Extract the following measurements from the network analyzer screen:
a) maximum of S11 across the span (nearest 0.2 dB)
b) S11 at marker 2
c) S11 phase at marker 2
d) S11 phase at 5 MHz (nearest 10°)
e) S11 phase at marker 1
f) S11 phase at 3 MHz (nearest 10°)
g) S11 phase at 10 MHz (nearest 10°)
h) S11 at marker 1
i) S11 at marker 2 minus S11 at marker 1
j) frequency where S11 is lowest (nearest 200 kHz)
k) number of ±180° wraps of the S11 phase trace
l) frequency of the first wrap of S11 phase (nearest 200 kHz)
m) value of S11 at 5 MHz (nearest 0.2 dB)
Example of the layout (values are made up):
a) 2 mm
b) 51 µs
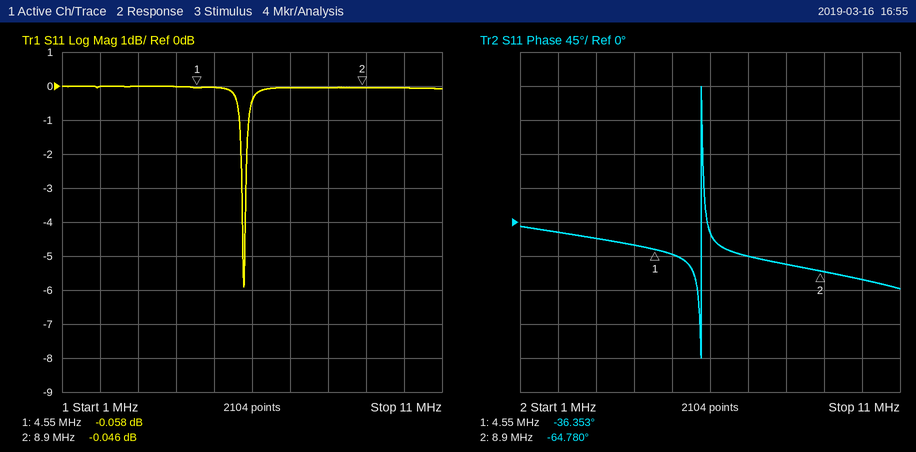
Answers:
a) 0.0 dB
b) -0.046 dB
c) -64.780°
d) -40°
e) -36.353°
f) -20°
g) -80°
h) -0.058 dB
i) 0.012 dB
j) 5.8 MHz
k) 1
l) 5.8 MHz
m) 0.0 dB
